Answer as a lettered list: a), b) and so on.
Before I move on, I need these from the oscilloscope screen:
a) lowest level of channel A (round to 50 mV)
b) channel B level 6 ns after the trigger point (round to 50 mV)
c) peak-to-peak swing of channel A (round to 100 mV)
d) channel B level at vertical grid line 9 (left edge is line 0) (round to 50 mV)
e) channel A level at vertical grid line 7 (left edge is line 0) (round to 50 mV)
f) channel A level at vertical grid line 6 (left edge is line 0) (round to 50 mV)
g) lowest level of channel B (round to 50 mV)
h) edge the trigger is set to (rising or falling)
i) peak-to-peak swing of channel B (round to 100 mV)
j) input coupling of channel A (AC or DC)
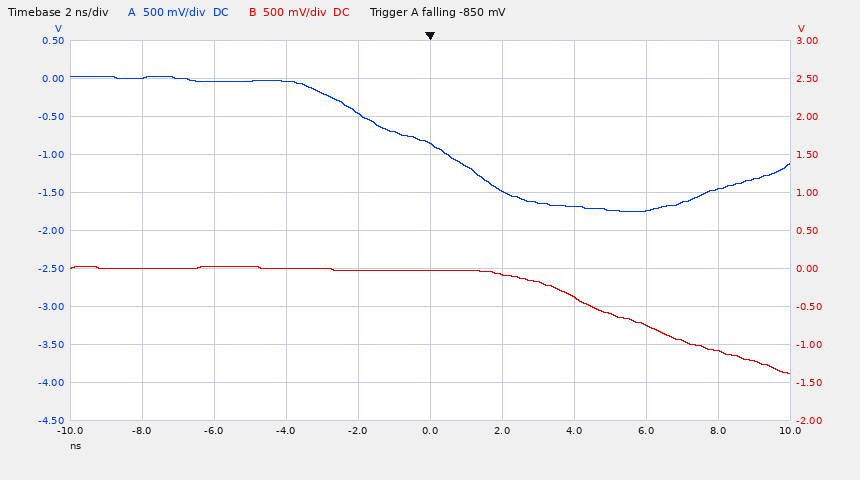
a) -1.75 V
b) -750 mV
c) 1.80 V
d) -1.10 V
e) -1.70 V
f) -1.50 V
g) -1.40 V
h) falling
i) 1.40 V
j) DC
